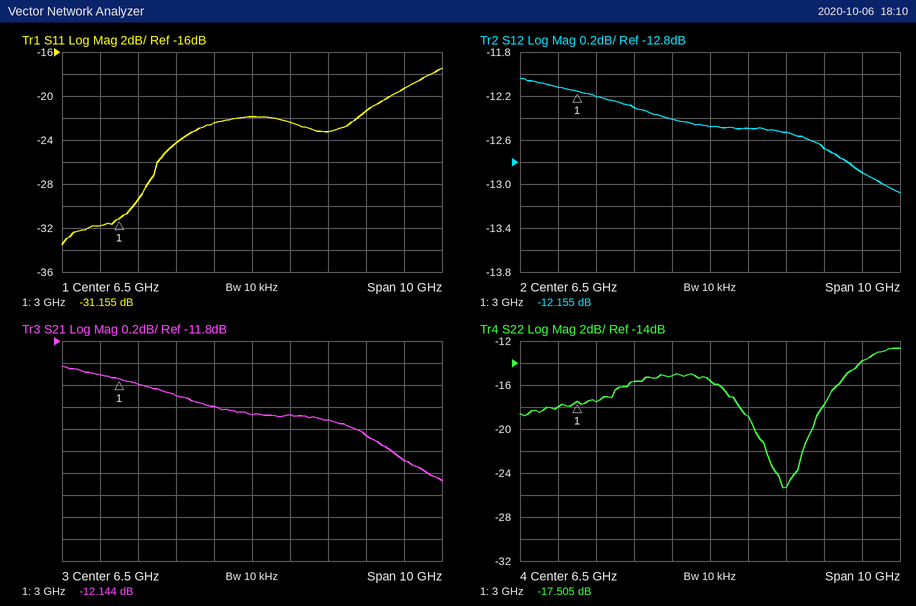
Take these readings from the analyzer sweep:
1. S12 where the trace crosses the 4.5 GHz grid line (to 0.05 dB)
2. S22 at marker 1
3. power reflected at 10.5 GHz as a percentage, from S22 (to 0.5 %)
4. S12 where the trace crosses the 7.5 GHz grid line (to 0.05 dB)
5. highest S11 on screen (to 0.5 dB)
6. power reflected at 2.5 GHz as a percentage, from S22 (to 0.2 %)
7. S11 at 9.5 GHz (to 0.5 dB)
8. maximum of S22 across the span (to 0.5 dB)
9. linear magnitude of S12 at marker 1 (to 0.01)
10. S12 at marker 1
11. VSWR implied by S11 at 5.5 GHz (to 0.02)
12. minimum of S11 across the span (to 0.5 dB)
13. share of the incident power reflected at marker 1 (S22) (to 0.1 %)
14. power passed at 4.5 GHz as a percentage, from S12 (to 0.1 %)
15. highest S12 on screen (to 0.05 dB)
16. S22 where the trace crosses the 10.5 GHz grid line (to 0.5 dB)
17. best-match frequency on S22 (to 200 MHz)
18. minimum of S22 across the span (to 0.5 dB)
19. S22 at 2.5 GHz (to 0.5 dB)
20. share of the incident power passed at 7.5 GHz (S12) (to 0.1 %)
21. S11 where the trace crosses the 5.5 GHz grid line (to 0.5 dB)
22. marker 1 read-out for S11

-12.30 dB
-17.505 dB
4.0 %
-12.50 dB
-17.5 dB
1.6 %
-21.5 dB
-12.5 dB
0.25
-12.155 dB
1.16
-33.5 dB
1.8 %
5.9 %
-12.05 dB
-14.0 dB
8.4 GHz
-25.5 dB
-18.0 dB
5.6 %
-22.5 dB
-31.155 dB
